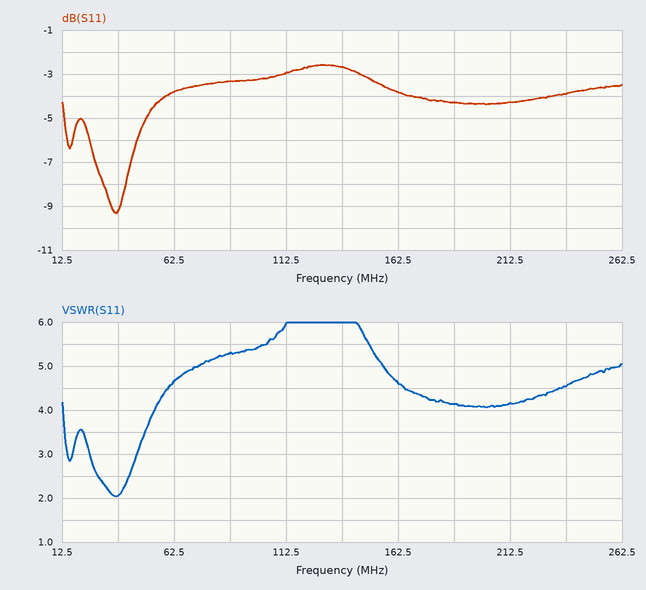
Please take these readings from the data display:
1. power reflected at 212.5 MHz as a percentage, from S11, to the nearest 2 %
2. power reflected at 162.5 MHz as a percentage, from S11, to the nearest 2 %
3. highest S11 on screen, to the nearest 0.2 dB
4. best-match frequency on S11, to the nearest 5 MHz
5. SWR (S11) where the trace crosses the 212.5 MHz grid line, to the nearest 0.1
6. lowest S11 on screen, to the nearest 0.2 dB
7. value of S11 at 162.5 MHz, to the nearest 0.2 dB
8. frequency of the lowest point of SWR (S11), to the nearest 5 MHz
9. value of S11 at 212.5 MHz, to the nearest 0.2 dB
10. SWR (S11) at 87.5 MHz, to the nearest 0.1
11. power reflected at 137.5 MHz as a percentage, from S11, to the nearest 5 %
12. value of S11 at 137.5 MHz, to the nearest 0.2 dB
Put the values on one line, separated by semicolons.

38 %; 42 %; -2.6 dB; 35 MHz; 4.2; -9.4 dB; -3.8 dB; 35 MHz; -4.2 dB; 5.3; 55 %; -2.6 dB
